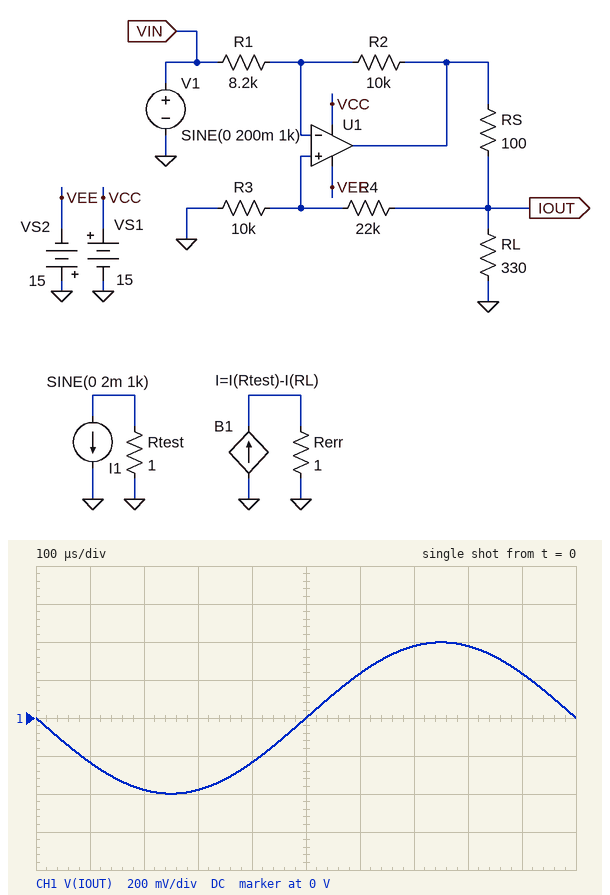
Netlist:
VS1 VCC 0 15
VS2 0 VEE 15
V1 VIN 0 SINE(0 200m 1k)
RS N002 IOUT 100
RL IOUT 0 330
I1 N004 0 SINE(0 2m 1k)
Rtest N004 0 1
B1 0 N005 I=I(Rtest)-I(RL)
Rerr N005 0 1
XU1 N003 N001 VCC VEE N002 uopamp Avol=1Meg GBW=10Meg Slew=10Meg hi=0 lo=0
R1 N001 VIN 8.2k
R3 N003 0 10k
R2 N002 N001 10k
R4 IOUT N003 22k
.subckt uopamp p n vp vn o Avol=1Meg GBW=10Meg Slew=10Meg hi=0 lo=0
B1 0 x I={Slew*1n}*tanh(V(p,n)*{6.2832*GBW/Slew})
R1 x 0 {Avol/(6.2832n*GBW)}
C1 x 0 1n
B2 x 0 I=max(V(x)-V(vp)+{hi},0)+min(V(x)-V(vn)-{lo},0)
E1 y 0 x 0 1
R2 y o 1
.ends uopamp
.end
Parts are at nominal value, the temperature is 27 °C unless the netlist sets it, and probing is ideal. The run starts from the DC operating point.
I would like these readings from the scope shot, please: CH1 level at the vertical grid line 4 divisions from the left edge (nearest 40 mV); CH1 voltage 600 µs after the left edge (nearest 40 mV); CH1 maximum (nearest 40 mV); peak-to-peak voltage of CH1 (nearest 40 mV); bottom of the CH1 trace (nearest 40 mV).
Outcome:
-240 mV
240 mV
400 mV
800 mV
-400 mV
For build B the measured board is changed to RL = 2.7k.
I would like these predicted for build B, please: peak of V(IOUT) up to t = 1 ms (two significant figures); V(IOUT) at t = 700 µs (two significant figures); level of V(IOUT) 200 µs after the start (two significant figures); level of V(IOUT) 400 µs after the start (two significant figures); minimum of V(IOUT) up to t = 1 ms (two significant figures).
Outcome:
700 mV
670 mV
-670 mV
-410 mV
-700 mV
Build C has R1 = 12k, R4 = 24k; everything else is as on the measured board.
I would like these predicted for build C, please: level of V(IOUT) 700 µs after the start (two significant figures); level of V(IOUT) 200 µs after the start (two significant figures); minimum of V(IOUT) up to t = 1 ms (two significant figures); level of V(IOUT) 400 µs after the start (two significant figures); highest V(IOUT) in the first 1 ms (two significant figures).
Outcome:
210 mV
-210 mV
-220 mV
-130 mV
220 mV
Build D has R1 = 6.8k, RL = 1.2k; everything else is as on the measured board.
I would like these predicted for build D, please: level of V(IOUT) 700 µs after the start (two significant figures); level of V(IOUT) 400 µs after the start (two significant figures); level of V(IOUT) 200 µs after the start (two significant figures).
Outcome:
890 mV
-550 mV
-890 mV
